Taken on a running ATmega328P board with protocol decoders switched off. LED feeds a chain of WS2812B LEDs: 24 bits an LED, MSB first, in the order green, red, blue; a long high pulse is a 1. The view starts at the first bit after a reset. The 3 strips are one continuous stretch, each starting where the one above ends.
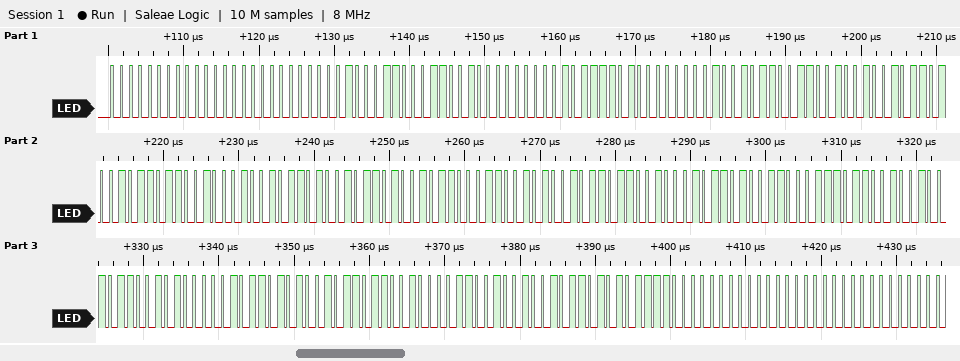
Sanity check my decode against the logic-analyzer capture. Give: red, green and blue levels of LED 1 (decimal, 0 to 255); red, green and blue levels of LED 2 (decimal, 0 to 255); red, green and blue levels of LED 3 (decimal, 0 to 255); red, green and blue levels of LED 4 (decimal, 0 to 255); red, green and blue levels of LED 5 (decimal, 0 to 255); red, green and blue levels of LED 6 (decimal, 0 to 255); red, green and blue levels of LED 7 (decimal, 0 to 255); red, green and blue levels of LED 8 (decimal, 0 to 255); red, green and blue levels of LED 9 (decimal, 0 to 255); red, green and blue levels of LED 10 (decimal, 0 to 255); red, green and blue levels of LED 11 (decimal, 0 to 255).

0, 0, 0
50, 70, 0
0, 189, 150
150, 100, 150
150, 200, 150
50, 150, 150
180, 200, 199
150, 100, 80
150, 90, 200
150, 100, 175
0, 0, 0
